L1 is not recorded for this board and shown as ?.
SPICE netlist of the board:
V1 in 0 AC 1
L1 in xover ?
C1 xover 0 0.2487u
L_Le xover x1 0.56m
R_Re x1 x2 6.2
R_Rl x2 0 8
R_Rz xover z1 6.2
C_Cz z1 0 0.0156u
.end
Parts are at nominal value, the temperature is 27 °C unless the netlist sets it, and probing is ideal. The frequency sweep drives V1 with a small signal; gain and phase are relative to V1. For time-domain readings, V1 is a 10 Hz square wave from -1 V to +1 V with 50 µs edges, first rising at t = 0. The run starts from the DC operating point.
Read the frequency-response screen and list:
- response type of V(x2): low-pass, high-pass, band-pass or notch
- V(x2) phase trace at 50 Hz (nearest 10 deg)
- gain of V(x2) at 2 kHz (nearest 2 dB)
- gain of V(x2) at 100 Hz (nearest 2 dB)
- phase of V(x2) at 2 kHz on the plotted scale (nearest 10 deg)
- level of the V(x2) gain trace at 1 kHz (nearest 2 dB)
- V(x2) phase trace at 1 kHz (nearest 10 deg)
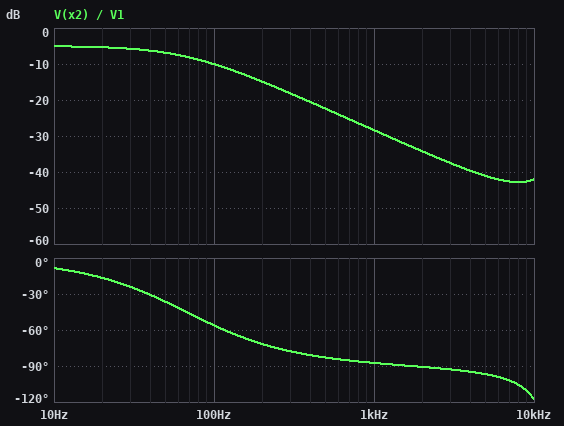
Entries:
low-pass
-40 deg
-34 dB
-10 dB
-90 deg
-28 dB
-90 deg
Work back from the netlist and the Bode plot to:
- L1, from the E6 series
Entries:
33 mH
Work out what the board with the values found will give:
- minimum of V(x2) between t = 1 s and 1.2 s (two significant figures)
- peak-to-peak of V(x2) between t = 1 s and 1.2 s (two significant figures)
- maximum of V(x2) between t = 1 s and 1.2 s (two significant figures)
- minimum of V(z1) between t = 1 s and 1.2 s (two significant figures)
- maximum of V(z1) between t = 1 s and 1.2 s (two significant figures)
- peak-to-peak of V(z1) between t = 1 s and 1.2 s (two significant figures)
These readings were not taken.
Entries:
-560 mV
1.1 V
560 mV
-1.0 V
1.0 V
2.0 V
